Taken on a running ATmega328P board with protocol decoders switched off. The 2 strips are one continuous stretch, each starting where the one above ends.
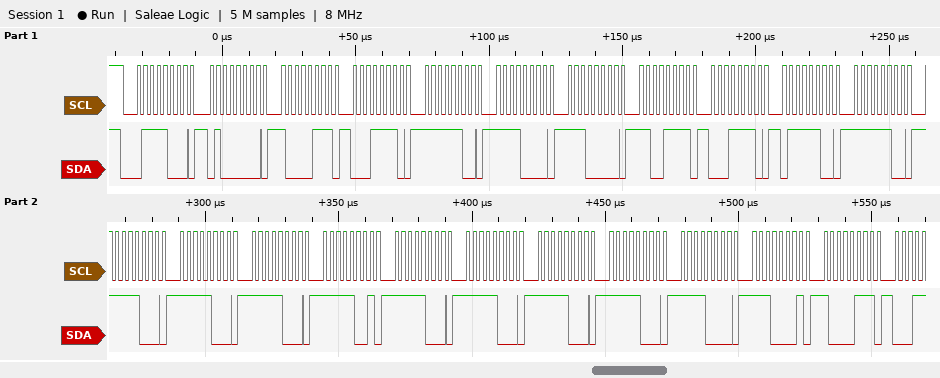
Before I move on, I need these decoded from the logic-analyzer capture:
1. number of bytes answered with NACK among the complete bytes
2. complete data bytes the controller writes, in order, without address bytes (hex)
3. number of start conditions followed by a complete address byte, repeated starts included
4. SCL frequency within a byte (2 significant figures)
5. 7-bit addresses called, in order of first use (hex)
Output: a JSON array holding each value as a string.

["0", "40 87 1E FC F0 E0 CF 1E 7C FC F8 F8 F8 F9 F8 F8 F8 F8 F0 E1 87", "1", "400 kHz", "0x3C"]
